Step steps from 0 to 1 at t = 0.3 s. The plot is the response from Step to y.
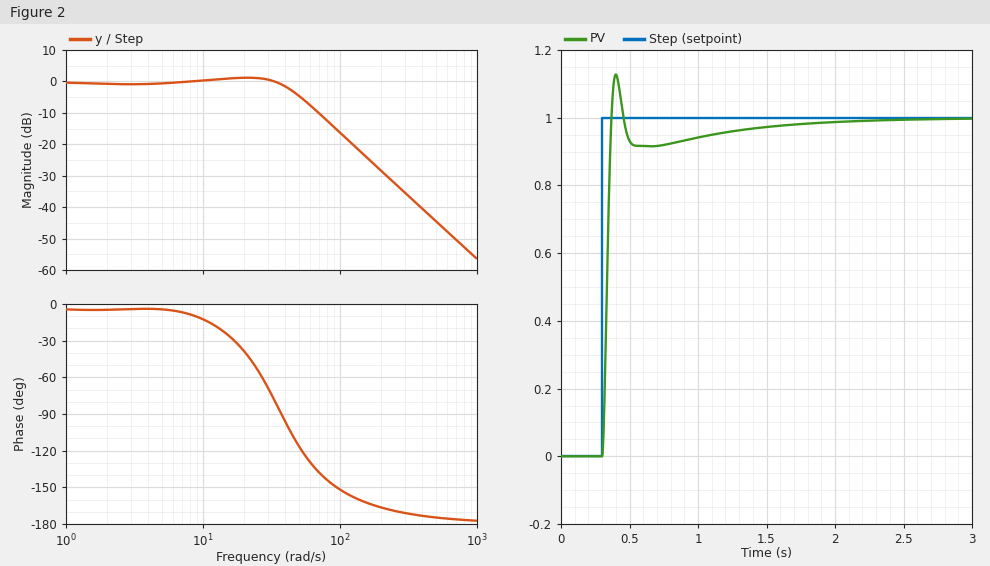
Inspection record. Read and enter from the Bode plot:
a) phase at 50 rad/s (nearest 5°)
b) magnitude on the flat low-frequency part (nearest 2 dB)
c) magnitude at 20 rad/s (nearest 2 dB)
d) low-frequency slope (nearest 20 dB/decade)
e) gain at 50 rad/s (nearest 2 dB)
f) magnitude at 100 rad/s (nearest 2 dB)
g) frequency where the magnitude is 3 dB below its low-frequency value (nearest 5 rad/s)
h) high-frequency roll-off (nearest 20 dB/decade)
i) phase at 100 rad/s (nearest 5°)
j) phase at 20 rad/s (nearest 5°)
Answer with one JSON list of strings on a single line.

["-115°", "0 dB", "2 dB", "0 dB/decade", "-4 dB", "-16 dB", "45 rad/s", "-40 dB/decade", "-150°", "-40°"]
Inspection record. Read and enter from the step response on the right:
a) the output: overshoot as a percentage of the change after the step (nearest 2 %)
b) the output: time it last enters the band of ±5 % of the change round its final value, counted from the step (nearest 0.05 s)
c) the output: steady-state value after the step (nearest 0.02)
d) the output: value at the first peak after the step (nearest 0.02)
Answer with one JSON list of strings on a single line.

["12 %", "0.80 s", "1.00", "1.12"]
